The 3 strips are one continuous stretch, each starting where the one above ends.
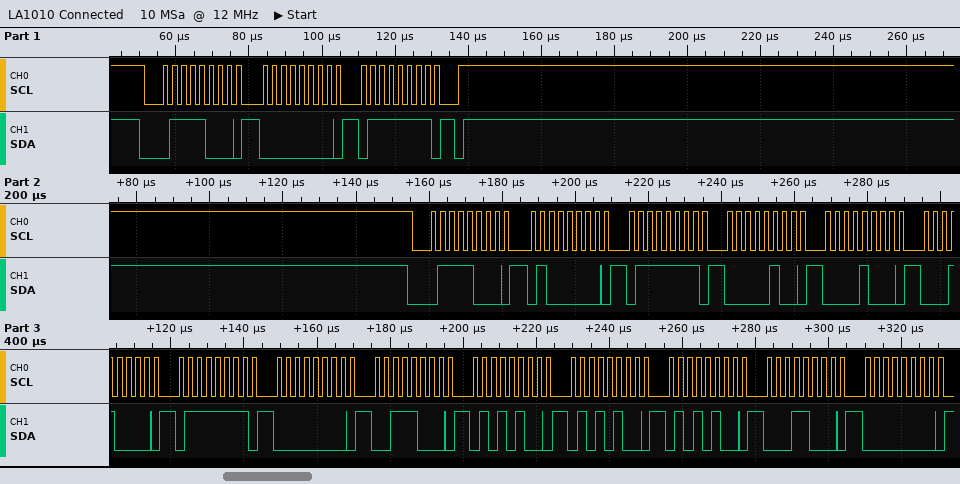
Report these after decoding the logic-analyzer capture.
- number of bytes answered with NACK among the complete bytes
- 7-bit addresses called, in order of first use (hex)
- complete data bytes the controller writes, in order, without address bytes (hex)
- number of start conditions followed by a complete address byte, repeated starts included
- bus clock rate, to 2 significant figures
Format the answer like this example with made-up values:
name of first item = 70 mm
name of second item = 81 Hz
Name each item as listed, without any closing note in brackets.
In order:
number of bytes answered with NACK among the complete bytes = 0
7-bit addresses called, in order of first use = 0x3C
complete data bytes the controller writes, in order, without address bytes = 00 7F 40 7F 04 08 10 7F 00 38 54 54 54 18 00
number of start conditions followed by a complete address byte, repeated starts included = 2
bus clock rate, to 2 significant figures = 400 kHz
